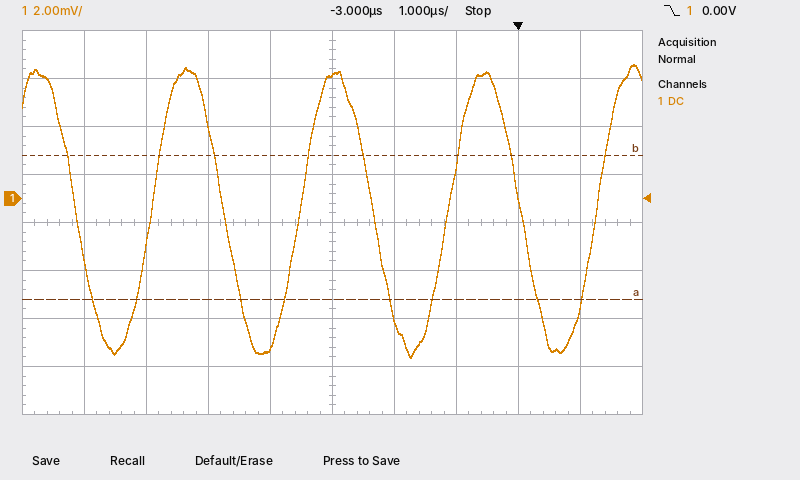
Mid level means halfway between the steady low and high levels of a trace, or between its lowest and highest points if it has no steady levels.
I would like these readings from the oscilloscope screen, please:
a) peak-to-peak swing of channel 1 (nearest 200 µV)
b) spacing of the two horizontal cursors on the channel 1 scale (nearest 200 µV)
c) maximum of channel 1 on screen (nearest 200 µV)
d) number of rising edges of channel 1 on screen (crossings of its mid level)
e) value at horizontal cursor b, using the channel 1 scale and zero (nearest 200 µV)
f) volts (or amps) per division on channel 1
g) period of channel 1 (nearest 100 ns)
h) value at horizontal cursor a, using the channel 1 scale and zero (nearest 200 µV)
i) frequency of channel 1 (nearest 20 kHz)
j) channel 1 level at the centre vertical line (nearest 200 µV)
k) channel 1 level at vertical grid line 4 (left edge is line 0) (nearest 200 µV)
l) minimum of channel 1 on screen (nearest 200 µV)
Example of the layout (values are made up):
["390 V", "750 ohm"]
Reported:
["12.2 mV", "6.0 mV", "5.6 mV", "4", "1.8 mV", "2 mV", "2.4 µs", "-4.2 mV", "420 kHz", "5.2 mV", "-6.2 mV", "-6.6 mV"]
